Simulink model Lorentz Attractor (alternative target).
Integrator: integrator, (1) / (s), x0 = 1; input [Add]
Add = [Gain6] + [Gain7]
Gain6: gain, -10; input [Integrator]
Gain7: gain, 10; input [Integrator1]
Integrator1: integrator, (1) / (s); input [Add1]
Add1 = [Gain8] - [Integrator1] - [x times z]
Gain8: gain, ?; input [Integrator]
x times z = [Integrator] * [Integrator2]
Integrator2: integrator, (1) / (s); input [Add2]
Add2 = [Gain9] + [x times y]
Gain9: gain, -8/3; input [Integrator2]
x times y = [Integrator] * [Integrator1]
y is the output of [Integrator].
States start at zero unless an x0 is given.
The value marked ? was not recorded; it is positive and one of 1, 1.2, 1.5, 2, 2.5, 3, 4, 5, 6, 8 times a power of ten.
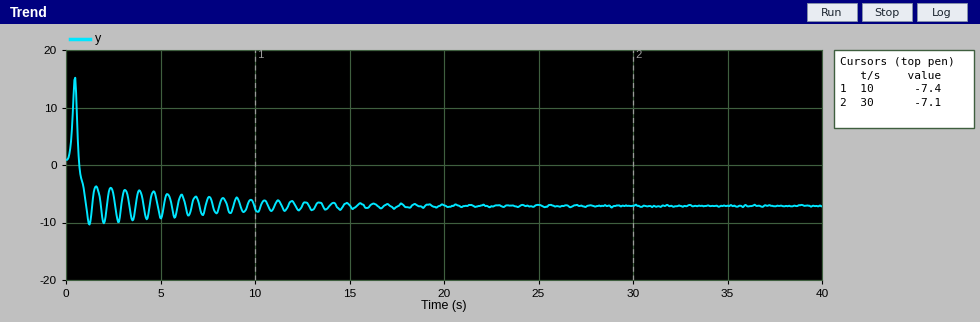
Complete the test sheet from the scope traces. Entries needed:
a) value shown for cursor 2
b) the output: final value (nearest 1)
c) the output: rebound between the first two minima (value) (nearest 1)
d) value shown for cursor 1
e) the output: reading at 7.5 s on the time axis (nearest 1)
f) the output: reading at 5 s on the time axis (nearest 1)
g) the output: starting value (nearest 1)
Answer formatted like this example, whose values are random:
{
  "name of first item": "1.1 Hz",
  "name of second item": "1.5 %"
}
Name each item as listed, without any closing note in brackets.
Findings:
{
  "value shown for cursor 2": "-7.1",
  "the output: final value": "-7",
  "the output: rebound between the first two minima (value)": "-4",
  "value shown for cursor 1": "-7.4",
  "the output: reading at 7.5 s on the time axis": "-6",
  "the output: reading at 5 s on the time axis": "-9",
  "the output: starting value": "1"
}
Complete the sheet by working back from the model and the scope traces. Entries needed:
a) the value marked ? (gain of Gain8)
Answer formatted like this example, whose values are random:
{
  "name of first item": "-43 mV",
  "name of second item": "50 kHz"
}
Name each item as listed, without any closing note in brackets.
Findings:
{
  "the value marked ?": "20"
}
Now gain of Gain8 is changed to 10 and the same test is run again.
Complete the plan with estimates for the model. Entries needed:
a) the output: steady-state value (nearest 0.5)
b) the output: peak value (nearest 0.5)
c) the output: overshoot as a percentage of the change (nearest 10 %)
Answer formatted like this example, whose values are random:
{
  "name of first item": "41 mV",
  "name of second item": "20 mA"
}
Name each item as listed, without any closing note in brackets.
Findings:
{
  "the output: steady-state value": "5.0",
  "the output: peak value": "8.5",
  "the output: overshoot as a percentage of the change": "100 %"
}
